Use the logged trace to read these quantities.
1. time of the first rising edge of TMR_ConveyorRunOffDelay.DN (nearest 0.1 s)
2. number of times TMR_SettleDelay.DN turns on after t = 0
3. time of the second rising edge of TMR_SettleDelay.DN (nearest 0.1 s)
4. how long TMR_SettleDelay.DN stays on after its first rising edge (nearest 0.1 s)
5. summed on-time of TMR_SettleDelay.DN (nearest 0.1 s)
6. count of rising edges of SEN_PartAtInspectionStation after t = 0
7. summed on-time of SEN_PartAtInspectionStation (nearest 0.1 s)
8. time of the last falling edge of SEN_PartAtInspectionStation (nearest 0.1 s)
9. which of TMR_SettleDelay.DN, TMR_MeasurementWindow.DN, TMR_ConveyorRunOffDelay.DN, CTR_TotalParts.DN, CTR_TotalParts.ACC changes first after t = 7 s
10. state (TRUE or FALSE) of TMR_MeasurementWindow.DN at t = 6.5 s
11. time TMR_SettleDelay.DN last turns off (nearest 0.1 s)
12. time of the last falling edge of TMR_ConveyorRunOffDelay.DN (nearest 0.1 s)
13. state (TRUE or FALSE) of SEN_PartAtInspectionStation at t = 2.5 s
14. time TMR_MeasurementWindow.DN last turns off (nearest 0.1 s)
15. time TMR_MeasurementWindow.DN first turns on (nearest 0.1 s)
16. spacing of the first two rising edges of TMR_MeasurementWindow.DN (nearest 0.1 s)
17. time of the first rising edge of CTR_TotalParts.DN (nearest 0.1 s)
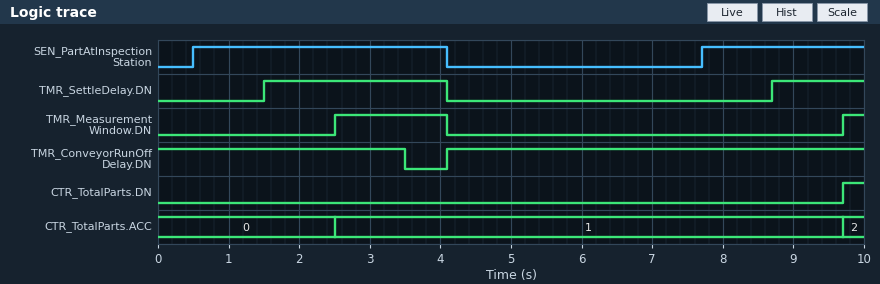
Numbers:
4.1 s
2
8.7 s
2.6 s
3.9 s
2
5.9 s
4.1 s
TMR_SettleDelay.DN
FALSE
4.1 s
3.5 s
TRUE
4.1 s
2.5 s
7.2 s
9.7 s
